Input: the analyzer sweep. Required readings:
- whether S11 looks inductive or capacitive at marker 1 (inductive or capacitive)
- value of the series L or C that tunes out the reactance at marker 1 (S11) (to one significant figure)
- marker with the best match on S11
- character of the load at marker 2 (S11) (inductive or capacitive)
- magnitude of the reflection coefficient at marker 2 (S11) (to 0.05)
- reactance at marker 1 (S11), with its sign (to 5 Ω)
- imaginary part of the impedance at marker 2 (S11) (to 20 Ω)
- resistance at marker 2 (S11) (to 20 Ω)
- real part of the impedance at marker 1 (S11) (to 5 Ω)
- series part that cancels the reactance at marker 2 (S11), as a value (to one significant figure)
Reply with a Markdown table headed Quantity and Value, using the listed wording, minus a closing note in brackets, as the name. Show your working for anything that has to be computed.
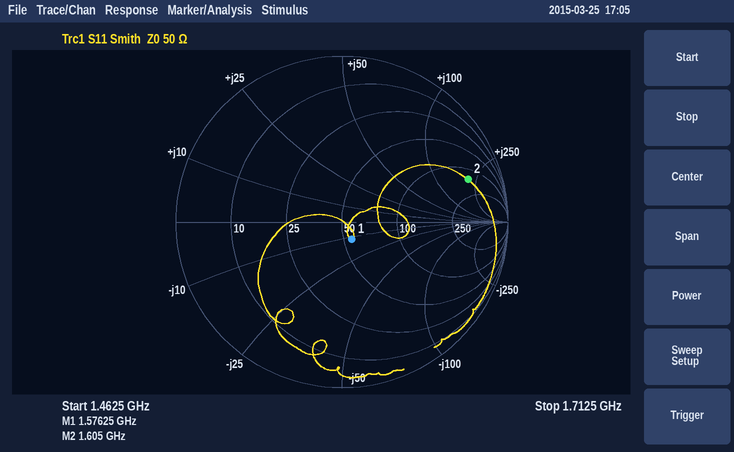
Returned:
| Quantity | Value |
|---|---|
| whether S11 looks inductive or capacitive at marker 1 | capacitive |
| value of the series L or C that tunes out the reactance at marker 1 (S11) | L = 10 Ω/(2π × 1.57625 GHz) ≈ 1 nH |
| marker with the best match on S11 | marker 1 |
| character of the load at marker 2 (S11) | inductive |
| magnitude of the reflection coefficient at marker 2 (S11) | 0.80 |
| reactance at marker 1 (S11), with its sign | -10 Ω |
| imaginary part of the impedance at marker 2 (S11) | +200 Ω |
| resistance at marker 2 (S11) | 140 Ω |
| real part of the impedance at marker 1 (S11) | 55 Ω |
| series part that cancels the reactance at marker 2 (S11), as a value | C = 1/(2π × 1.605 GHz × 200 Ω) ≈ 496 fF, so 500 fF to one significant figure |
